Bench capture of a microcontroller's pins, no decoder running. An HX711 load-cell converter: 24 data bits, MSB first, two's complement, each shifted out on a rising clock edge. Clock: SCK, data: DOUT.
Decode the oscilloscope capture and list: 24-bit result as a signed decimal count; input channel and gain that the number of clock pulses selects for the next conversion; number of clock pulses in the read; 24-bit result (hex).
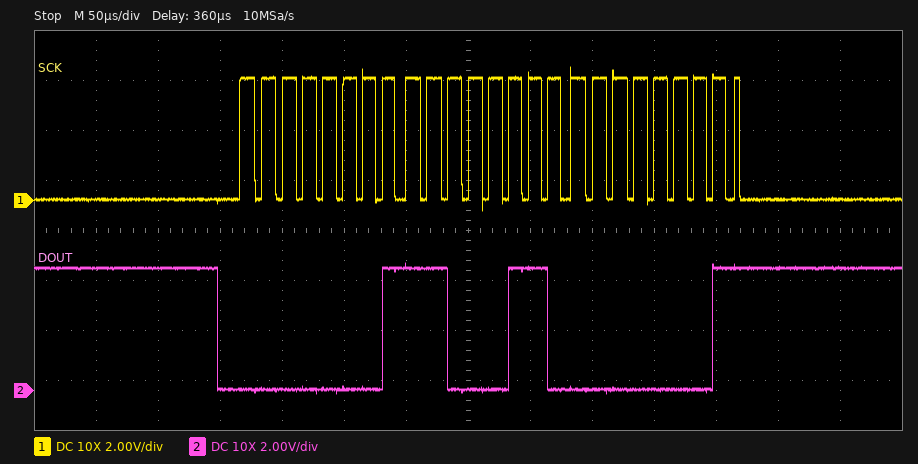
116225
channel A, gain 128
25
0x01C601
